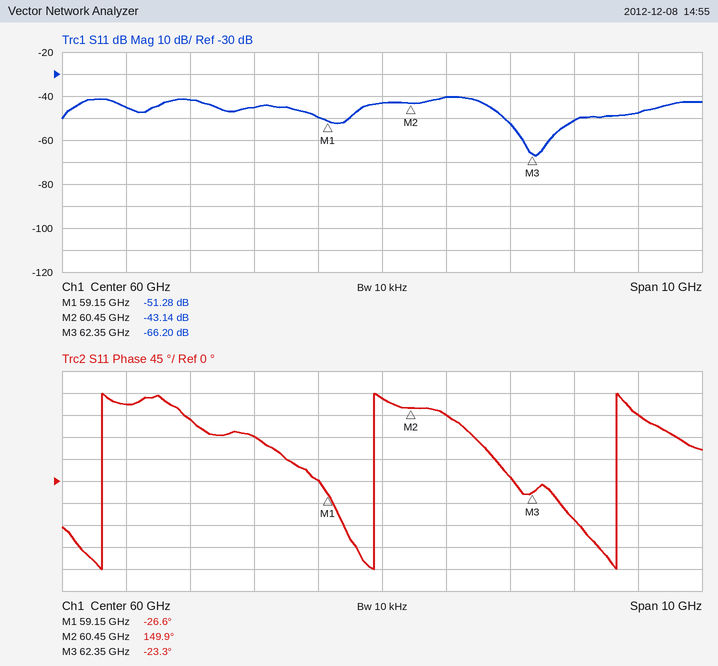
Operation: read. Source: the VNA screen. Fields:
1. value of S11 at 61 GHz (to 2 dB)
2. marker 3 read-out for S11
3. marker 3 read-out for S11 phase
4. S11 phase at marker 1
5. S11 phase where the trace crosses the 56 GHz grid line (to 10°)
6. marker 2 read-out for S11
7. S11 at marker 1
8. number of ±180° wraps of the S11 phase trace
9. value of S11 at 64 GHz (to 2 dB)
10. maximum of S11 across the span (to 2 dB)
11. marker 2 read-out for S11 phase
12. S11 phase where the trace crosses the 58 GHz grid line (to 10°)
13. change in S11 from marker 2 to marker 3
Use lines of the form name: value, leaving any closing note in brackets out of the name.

value of S11 at 61 GHz: -40 dB
marker 3 read-out for S11: -66.20 dB
marker 3 read-out for S11 phase: -23.3°
S11 phase at marker 1: -26.6°
S11 phase where the trace crosses the 56 GHz grid line: 160°
marker 2 read-out for S11: -43.14 dB
S11 at marker 1: -51.28 dB
number of ±180° wraps of the S11 phase trace: 3
value of S11 at 64 GHz: -48 dB
maximum of S11 across the span: -40 dB
marker 2 read-out for S11 phase: 149.9°
S11 phase where the trace crosses the 58 GHz grid line: 90°
change in S11 from marker 2 to marker 3: -23.06 dB
